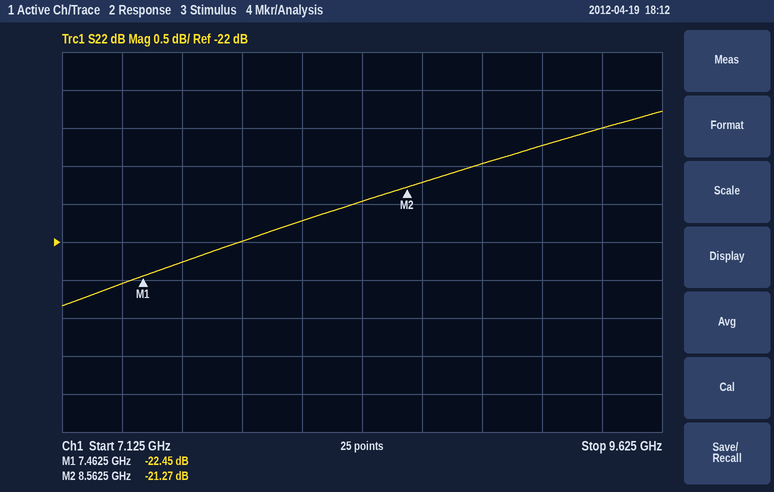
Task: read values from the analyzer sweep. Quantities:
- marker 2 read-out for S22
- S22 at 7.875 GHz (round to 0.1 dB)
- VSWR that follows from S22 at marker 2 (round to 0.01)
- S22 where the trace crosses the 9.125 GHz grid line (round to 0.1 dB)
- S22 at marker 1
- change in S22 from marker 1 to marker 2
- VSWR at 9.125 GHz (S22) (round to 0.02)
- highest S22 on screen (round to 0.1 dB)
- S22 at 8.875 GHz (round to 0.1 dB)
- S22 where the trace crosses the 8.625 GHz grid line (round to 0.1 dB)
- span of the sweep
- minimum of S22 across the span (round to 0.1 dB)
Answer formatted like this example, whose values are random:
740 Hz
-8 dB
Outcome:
-21.27 dB
-22.0 dB
1.19
-20.7 dB
-22.45 dB
1.18 dB
1.20
-20.3 dB
-21.0 dB
-21.2 dB
2.5 GHz
-22.8 dB
